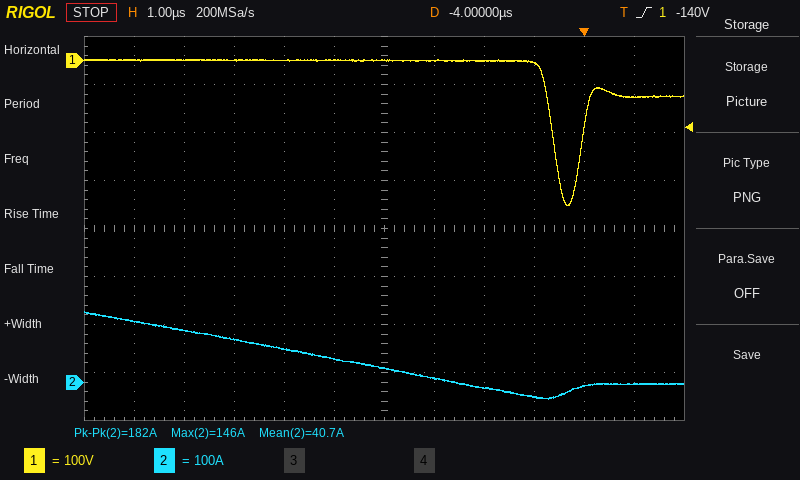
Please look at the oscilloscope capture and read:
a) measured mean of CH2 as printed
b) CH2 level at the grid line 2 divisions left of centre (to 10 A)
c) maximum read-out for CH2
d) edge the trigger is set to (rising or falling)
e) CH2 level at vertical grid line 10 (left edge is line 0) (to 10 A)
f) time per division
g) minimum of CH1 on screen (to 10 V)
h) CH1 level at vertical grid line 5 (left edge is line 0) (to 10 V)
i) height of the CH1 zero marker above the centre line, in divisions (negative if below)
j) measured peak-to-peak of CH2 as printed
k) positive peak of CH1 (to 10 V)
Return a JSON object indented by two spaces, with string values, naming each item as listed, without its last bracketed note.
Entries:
{
  "measured mean of CH2 as printed": "40.7 A",
  "CH2 level at the grid line 2 divisions left of centre": "70 A",
  "maximum read-out for CH2": "146 A",
  "edge the trigger is set to": "rising",
  "CH2 level at vertical grid line 10 (left edge is line 0)": "-10 A",
  "time per division": "1 µs",
  "minimum of CH1 on screen": "-300 V",
  "CH1 level at vertical grid line 5 (left edge is line 0)": "0 V",
  "height of the CH1 zero marker above the centre line, in divisions": "+3.5 div",
  "measured peak-to-peak of CH2 as printed": "182 A",
  "positive peak of CH1": "0 V"
}
